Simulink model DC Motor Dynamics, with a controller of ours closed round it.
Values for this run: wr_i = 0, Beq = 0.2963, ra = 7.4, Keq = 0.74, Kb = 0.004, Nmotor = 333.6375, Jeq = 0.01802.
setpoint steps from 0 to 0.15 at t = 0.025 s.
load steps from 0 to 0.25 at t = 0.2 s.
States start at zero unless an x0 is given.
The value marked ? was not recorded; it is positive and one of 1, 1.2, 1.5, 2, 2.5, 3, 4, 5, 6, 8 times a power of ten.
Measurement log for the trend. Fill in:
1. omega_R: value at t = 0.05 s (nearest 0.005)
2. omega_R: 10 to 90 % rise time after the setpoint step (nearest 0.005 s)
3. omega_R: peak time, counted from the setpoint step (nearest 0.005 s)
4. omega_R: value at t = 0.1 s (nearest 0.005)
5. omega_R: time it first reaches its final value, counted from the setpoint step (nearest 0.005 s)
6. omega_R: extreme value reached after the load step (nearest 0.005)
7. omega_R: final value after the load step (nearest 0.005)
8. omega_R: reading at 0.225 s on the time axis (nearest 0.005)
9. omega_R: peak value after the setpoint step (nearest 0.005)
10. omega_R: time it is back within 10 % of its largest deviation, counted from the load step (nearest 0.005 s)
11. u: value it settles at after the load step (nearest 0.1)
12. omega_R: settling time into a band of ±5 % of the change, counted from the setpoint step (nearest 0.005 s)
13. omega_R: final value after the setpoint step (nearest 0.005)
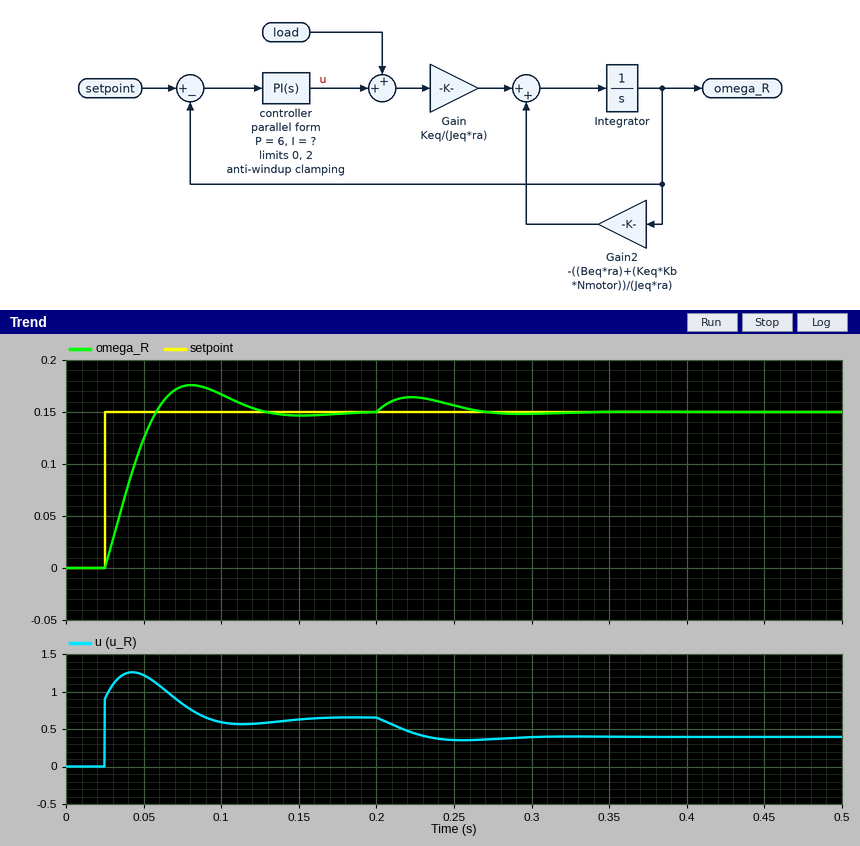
0.125
0.025 s
0.055 s
0.165
0.035 s
0.165
0.150
0.165
0.175
0.110 s
0.4
0.090 s
0.150
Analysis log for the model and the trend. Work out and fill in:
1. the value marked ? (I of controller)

500
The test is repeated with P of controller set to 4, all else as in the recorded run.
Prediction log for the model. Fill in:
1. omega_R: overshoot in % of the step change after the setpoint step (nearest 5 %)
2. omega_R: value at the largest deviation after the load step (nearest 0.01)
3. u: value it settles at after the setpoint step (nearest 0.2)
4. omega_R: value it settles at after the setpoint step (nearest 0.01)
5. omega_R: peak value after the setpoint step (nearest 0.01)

25 %
0.17
0.6
0.15
0.19
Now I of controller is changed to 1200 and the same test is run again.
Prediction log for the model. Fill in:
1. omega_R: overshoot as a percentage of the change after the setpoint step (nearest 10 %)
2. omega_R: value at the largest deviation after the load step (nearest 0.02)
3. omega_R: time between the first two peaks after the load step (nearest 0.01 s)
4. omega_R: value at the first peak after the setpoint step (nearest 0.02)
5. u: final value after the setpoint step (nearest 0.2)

30 %
0.16
0.08 s
0.20
0.6
